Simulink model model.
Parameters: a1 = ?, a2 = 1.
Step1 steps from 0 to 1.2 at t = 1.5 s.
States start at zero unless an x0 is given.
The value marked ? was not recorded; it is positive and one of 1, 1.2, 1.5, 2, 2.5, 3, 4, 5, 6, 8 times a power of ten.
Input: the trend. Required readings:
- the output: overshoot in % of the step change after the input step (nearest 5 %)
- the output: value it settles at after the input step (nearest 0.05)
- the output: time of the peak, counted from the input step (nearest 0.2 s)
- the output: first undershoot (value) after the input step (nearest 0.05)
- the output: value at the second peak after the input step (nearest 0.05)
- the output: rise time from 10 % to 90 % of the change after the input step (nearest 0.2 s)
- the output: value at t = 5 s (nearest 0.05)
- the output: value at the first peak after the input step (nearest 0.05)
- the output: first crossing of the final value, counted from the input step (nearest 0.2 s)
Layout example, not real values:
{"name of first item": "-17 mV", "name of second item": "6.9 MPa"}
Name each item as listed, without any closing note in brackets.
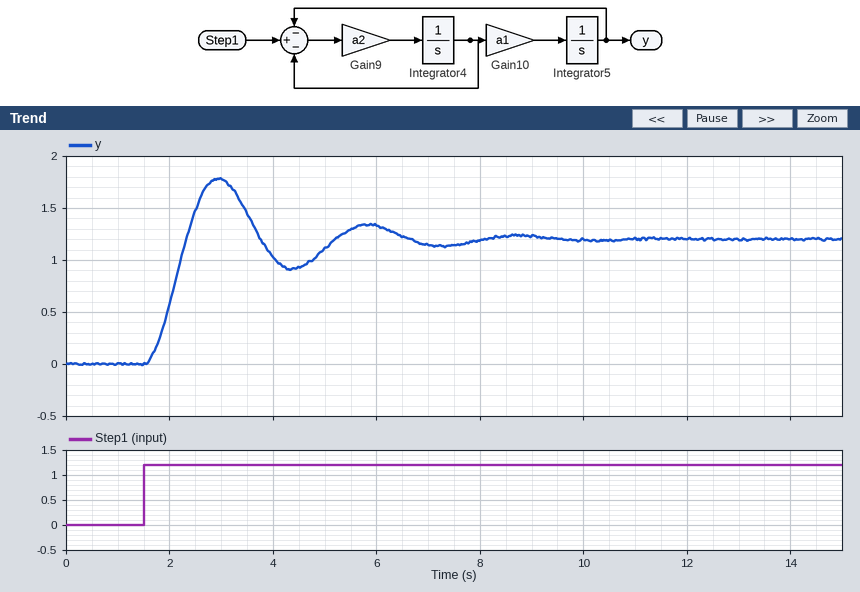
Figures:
{"the output: overshoot in % of the step change after the input step": "50 %", "the output: value it settles at after the input step": "1.20", "the output: time of the peak, counted from the input step": "1.4 s", "the output: first undershoot (value) after the input step": "0.90", "the output: value at the second peak after the input step": "1.35", "the output: rise time from 10 % to 90 % of the change after the input step": "0.6 s", "the output: value at t = 5 s": "1.10", "the output: value at the first peak after the input step": "1.80", "the output: first crossing of the final value, counted from the input step": "0.8 s"}
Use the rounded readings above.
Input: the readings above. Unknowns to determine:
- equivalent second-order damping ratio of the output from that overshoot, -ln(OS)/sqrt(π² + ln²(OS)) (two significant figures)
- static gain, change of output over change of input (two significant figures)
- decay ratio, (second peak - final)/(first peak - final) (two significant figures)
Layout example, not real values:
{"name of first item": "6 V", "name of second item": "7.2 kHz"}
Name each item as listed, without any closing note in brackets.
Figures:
{"equivalent second-order damping ratio of the output from that overshoot, -ln(OS)/sqrt(π² + ln²(OS))": "0.22", "static gain, change of output over change of input": "1.0", "decay ratio, (second peak - final)/(first peak - final)": "0.25"}
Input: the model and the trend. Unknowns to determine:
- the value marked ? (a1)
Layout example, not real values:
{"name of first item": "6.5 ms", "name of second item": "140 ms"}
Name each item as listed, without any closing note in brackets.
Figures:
{"the value marked ?": "5"}
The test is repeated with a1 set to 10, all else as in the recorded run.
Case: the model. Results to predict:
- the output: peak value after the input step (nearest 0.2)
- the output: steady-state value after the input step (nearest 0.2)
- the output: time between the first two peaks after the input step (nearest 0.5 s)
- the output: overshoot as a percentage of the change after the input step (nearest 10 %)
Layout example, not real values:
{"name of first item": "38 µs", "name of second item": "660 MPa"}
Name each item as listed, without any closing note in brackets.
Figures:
{"the output: peak value after the input step": "2.0", "the output: steady-state value after the input step": "1.2", "the output: time between the first two peaks after the input step": "2.0 s", "the output: overshoot as a percentage of the change after the input step": "60 %"}
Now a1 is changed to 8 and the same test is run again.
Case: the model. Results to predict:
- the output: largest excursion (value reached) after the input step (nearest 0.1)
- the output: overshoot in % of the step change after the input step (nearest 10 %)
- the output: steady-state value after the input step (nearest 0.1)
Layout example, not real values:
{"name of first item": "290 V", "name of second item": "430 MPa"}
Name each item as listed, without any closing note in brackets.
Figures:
{"the output: largest excursion (value reached) after the input step": "1.9", "the output: overshoot in % of the step change after the input step": "60 %", "the output: steady-state value after the input step": "1.2"}
